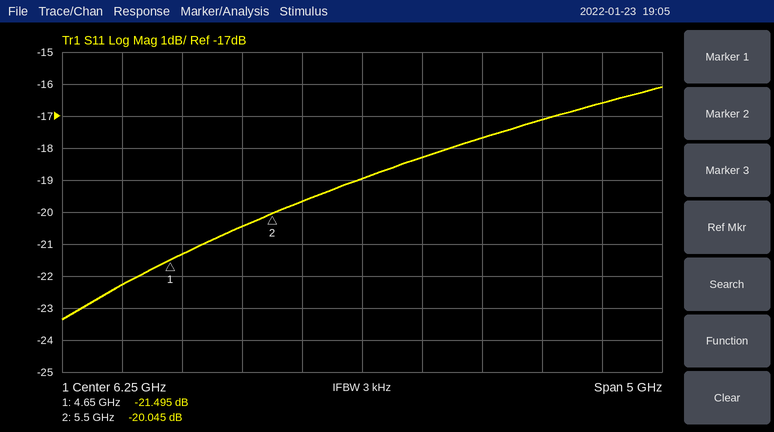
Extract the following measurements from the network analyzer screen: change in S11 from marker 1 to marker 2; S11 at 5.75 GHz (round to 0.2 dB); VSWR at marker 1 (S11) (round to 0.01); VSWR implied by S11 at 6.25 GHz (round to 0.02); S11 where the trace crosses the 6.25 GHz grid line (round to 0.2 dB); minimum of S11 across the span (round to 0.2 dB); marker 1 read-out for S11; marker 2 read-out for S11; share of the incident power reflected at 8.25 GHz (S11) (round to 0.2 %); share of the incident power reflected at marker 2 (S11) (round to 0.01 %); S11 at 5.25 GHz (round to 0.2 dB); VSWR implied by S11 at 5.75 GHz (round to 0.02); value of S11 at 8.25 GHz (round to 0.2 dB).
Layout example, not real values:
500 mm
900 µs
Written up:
1.450 dB
-19.6 dB
1.18
1.26
-19.0 dB
-23.4 dB
-21.495 dB
-20.045 dB
2.2 %
0.99 %
-20.4 dB
1.24
-16.6 dB
